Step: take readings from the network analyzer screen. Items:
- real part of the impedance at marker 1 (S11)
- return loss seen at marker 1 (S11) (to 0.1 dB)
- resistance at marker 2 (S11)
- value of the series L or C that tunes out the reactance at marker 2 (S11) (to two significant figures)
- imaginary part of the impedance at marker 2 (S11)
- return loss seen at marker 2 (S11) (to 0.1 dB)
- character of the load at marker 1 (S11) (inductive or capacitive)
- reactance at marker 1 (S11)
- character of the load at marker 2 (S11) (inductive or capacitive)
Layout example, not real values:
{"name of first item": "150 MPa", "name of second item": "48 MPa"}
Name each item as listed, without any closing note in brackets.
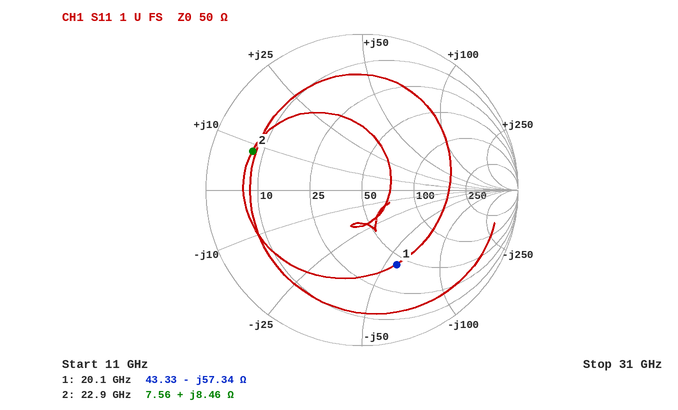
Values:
{"real part of the impedance at marker 1": "43.33 Ω", "return loss seen at marker 1 (S11)": "5.6 dB", "resistance at marker 2": "7.56 Ω", "value of the series L or C that tunes out the reactance at marker 2 (S11)": "820 fF", "imaginary part of the impedance at marker 2": "+8.46 Ω", "return loss seen at marker 2 (S11)": "2.6 dB", "character of the load at marker 1 (S11)": "capacitive", "reactance at marker 1": "-57.34 Ω", "character of the load at marker 2 (S11)": "inductive"}
